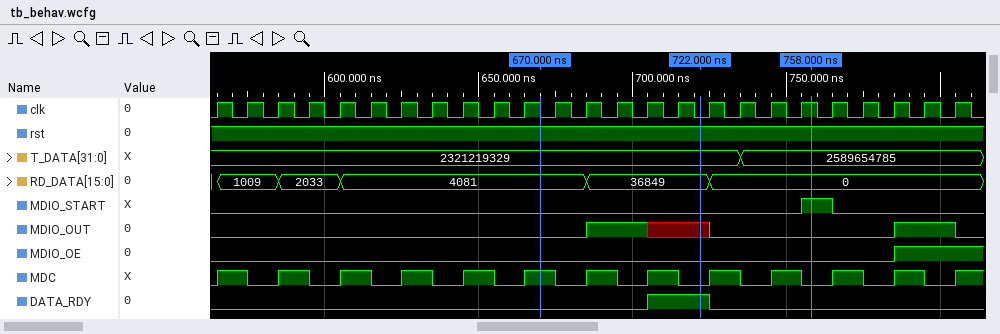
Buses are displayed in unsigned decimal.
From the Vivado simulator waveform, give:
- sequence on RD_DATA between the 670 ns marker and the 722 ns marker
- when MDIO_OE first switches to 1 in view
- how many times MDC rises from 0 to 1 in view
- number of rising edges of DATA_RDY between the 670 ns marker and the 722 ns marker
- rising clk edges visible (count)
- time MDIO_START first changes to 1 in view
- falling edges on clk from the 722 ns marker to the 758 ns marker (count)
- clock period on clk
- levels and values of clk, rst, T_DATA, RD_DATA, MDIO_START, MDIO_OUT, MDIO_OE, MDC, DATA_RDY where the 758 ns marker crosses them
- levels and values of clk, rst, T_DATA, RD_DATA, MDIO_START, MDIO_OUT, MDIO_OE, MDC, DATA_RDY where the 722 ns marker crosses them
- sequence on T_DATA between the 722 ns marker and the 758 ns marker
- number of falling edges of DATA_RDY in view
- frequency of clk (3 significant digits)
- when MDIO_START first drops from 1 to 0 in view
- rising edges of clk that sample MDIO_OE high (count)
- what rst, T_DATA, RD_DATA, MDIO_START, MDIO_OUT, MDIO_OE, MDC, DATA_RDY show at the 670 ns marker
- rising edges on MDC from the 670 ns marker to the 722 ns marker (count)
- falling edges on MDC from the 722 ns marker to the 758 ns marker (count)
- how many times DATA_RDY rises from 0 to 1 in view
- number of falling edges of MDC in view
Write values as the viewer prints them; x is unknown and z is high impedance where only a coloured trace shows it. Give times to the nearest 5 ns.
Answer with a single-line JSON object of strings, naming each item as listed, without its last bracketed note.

{"sequence on RD_DATA between the 670 ns marker and the 722 ns marker": "4081, 36849", "when MDIO_OE first switches to 1 in view": "785 ns", "how many times MDC rises from 0 to 1 in view": "13", "number of rising edges of DATA_RDY between the 670 ns marker and the 722 ns marker": "1", "rising clk edges visible": "25", "time MDIO_START first changes to 1 in view": "755 ns", "falling edges on clk from the 722 ns marker to the 758 ns marker": "3", "clock period on clk": "10 ns", "levels and values of clk, rst, T_DATA, RD_DATA, MDIO_START, MDIO_OUT, MDIO_OE, MDC, DATA_RDY where the 758 ns marker crosses them": "clk=1, rst=1, T_DATA=2589654785, RD_DATA=0, MDIO_START=1, MDIO_OUT=0, MDIO_OE=0, MDC=0, DATA_RDY=0", "levels and values of clk, rst, T_DATA, RD_DATA, MDIO_START, MDIO_OUT, MDIO_OE, MDC, DATA_RDY where the 722 ns marker crosses them": "clk=0, rst=1, T_DATA=2321219329, RD_DATA=36849, MDIO_START=0, MDIO_OUT=x, MDIO_OE=0, MDC=0, DATA_RDY=1", "sequence on T_DATA between the 722 ns marker and the 758 ns marker": "2321219329, 2589654785", "number of falling edges of DATA_RDY in view": "1", "frequency of clk": "100 MHz", "when MDIO_START first drops from 1 to 0 in view": "765 ns", "rising edges of clk that sample MDIO_OE high": "2", "what rst, T_DATA, RD_DATA, MDIO_START, MDIO_OUT, MDIO_OE, MDC, DATA_RDY show at the 670 ns marker": "rst=1, T_DATA=2321219329, RD_DATA=4081, MDIO_START=0, MDIO_OUT=0, MDIO_OE=0, MDC=1, DATA_RDY=0", "rising edges on MDC from the 670 ns marker to the 722 ns marker": "2", "falling edges on MDC from the 722 ns marker to the 758 ns marker": "2", "how many times DATA_RDY rises from 0 to 1 in view": "1", "number of falling edges of MDC in view": "12"}
